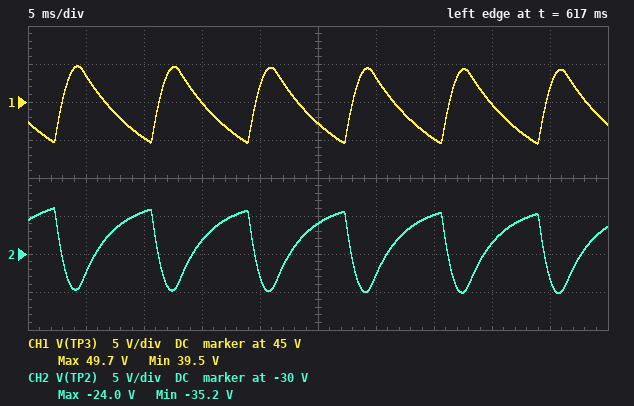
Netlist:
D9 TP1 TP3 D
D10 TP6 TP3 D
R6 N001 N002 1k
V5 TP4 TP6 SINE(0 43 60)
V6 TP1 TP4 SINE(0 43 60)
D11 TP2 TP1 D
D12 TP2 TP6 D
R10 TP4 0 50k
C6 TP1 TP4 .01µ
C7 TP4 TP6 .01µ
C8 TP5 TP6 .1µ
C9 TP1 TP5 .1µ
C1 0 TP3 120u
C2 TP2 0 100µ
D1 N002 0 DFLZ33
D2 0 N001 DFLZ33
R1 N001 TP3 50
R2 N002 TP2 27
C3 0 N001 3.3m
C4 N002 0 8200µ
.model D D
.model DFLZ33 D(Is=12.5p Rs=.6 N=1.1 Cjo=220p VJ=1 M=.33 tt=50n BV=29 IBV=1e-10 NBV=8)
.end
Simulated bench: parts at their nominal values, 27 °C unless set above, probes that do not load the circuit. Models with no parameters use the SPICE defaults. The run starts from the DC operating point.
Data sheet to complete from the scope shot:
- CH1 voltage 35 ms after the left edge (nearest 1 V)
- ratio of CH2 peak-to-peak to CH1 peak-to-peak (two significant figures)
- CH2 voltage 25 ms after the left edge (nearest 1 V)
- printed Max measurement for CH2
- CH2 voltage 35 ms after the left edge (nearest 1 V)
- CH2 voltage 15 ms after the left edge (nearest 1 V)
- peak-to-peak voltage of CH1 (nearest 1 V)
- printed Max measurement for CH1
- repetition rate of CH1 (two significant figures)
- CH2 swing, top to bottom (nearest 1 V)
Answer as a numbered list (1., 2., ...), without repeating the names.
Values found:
1. 40 V
2. 1.1
3. -26 V
4. -24.0 V
5. -25 V
6. -28 V
7. 10 V
8. 49.7 V
9. 120 Hz
10. 11 V
